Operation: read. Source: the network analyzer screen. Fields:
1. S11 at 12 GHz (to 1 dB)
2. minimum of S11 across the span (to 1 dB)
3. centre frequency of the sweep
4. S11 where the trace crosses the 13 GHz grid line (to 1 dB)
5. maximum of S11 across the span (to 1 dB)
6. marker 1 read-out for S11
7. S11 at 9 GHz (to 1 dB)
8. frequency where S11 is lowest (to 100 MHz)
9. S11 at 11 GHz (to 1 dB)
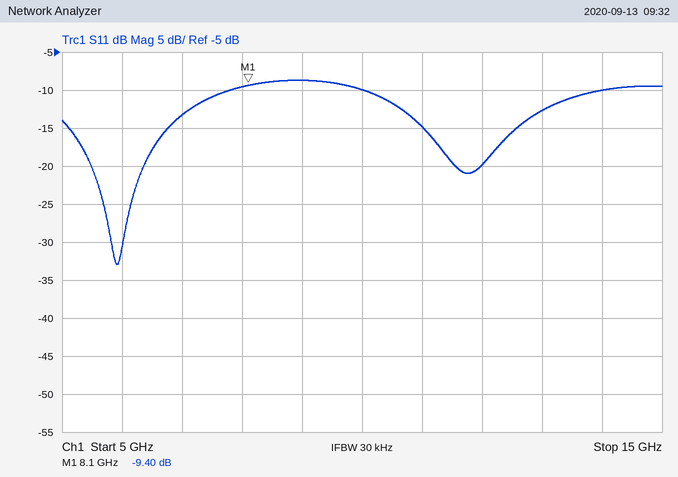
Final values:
-20 dB
-33 dB
10 GHz
-13 dB
-9 dB
-9.40 dB
-9 dB
5.9 GHz
-15 dB
